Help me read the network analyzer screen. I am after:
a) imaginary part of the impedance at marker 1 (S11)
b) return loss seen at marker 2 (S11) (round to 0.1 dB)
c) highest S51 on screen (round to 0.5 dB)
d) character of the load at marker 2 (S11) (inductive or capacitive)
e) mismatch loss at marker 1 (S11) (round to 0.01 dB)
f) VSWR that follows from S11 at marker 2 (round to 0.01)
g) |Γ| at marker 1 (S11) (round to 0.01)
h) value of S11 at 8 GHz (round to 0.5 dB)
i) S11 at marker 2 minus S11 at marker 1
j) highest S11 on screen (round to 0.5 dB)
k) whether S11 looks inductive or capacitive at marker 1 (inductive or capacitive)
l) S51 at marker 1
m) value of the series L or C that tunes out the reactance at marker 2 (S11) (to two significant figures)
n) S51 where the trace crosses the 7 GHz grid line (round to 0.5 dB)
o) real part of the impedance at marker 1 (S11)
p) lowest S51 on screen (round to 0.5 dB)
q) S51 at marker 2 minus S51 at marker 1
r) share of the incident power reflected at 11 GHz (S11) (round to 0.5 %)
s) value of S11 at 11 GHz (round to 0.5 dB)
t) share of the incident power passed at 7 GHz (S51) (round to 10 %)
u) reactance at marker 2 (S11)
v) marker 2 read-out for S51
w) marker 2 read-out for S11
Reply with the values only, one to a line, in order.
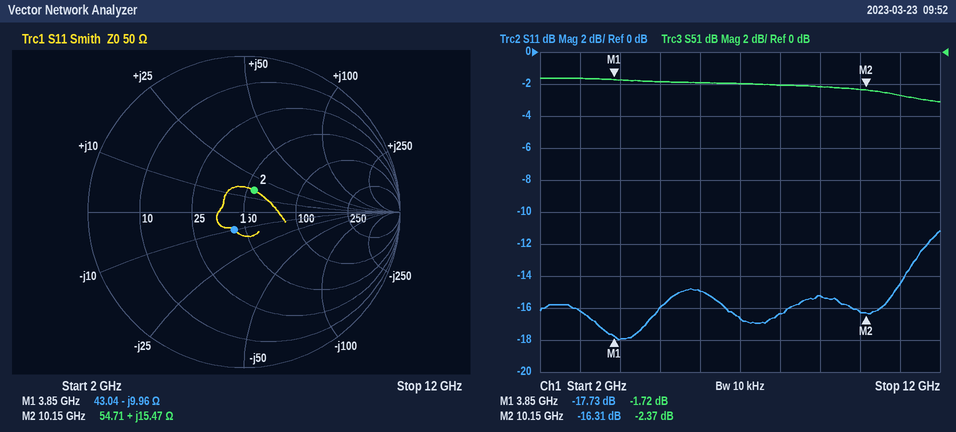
-9.96 Ω
16.3 dB
-1.5 dB
inductive
0.07 dB
1.36
0.13
-16.5 dB
1.42 dB
-11.0 dB
capacitive
-1.72 dB
1.0 pF
-2.0 dB
43.04 Ω
-3.0 dB
-0.65 dB
3.5 %
-14.5 dB
60 %
+15.47 Ω
-2.37 dB
-16.31 dB
